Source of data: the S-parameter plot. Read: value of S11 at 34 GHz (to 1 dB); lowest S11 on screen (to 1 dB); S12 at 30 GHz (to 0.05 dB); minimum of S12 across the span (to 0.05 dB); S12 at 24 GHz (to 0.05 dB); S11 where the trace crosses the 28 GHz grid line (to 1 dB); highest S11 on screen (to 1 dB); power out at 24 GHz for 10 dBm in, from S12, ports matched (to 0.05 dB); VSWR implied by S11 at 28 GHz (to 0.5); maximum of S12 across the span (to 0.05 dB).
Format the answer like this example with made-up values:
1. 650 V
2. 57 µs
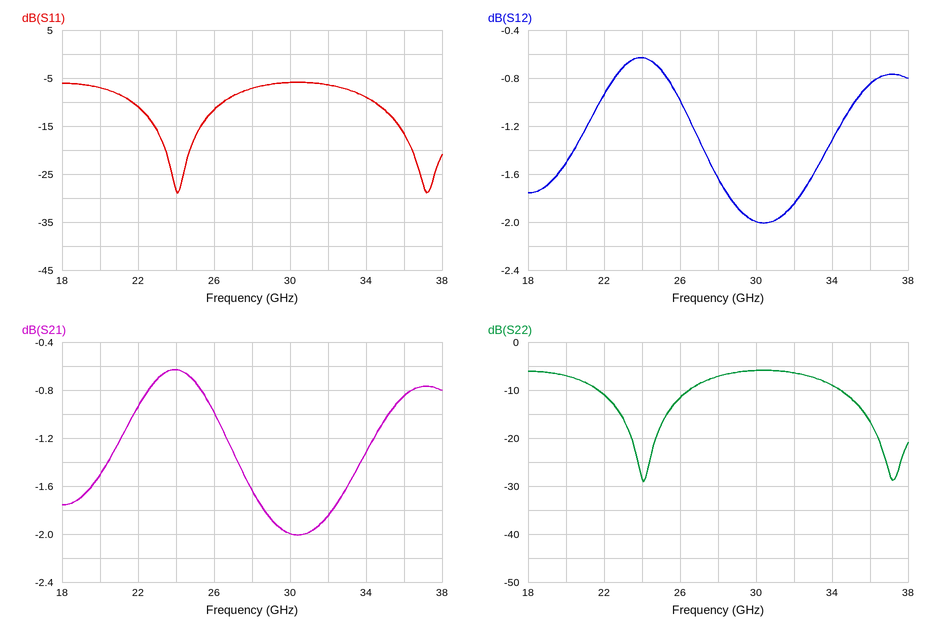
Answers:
1. -9 dB
2. -29 dB
3. -2.00 dB
4. -2.00 dB
5. -0.65 dB
6. -7 dB
7. -6 dB
8. 9.35 dBm
9. 2.5
10. -0.65 dB
